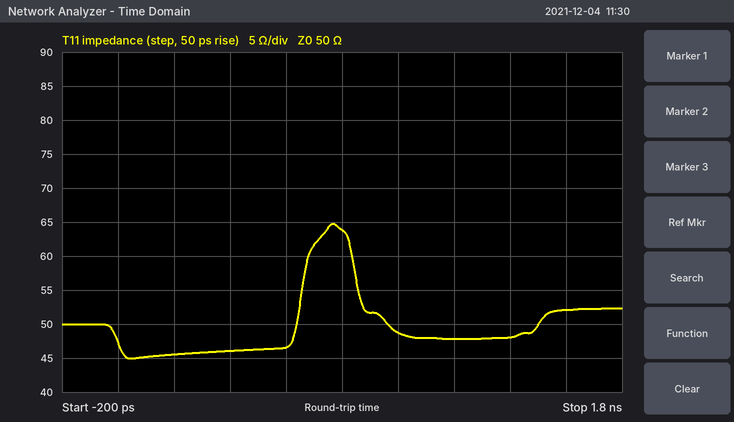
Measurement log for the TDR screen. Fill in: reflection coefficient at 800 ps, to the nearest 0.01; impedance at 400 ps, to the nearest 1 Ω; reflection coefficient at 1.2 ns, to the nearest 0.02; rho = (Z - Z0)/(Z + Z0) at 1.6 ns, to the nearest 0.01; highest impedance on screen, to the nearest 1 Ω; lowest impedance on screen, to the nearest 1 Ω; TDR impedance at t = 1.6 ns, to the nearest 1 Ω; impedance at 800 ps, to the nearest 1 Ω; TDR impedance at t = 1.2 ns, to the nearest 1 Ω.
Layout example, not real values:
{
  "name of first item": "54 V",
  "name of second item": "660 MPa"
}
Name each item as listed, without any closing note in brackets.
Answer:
{
  "reflection coefficient at 800 ps, to the nearest 0.01": "+0.12",
  "impedance at 400 ps, to the nearest 1 Ω": "46 Ω",
  "reflection coefficient at 1.2 ns, to the nearest 0.02": "-0.02",
  "rho = (Z - Z0)/(Z + Z0) at 1.6 ns, to the nearest 0.01": "+0.02",
  "highest impedance on screen, to the nearest 1 Ω": "65 Ω",
  "lowest impedance on screen, to the nearest 1 Ω": "45 Ω",
  "TDR impedance at t = 1.6 ns, to the nearest 1 Ω": "52 Ω",
  "impedance at 800 ps, to the nearest 1 Ω": "64 Ω",
  "TDR impedance at t = 1.2 ns, to the nearest 1 Ω": "48 Ω"
}
